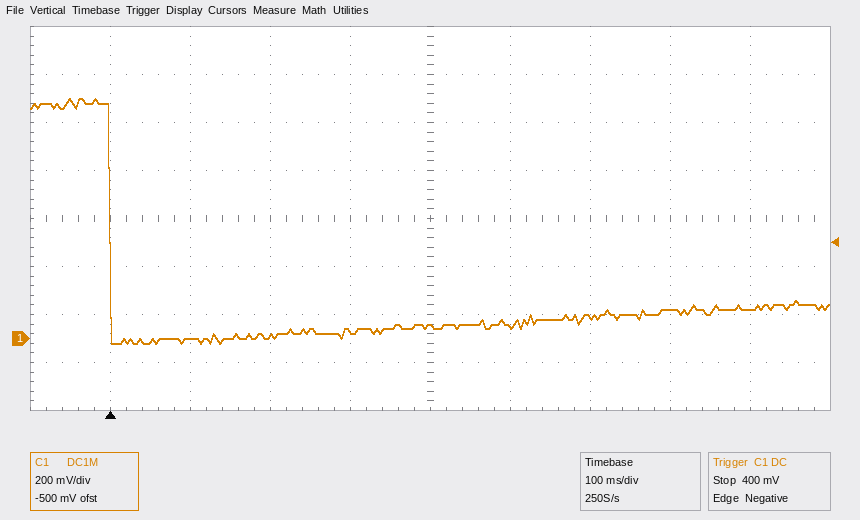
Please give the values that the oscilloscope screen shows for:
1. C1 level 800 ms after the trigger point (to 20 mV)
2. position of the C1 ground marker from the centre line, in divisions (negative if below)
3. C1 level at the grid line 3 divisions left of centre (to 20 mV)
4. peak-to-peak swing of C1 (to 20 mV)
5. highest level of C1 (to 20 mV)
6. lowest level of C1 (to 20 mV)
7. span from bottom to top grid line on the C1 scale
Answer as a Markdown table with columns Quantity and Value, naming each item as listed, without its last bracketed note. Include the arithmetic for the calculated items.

| Quantity | Value |
|---|---|
| C1 level 800 ms after the trigger point | 120 mV |
| position of the C1 ground marker from the centre line, in divisions | -2.5 div |
| C1 level at the grid line 3 divisions left of centre | 0 mV |
| peak-to-peak swing of C1 | 1.00 V − (-20 mV) = 1.02 V |
| highest level of C1 | 1.00 V |
| lowest level of C1 | -20 mV |
| span from bottom to top grid line on the C1 scale | 1.6 V |
